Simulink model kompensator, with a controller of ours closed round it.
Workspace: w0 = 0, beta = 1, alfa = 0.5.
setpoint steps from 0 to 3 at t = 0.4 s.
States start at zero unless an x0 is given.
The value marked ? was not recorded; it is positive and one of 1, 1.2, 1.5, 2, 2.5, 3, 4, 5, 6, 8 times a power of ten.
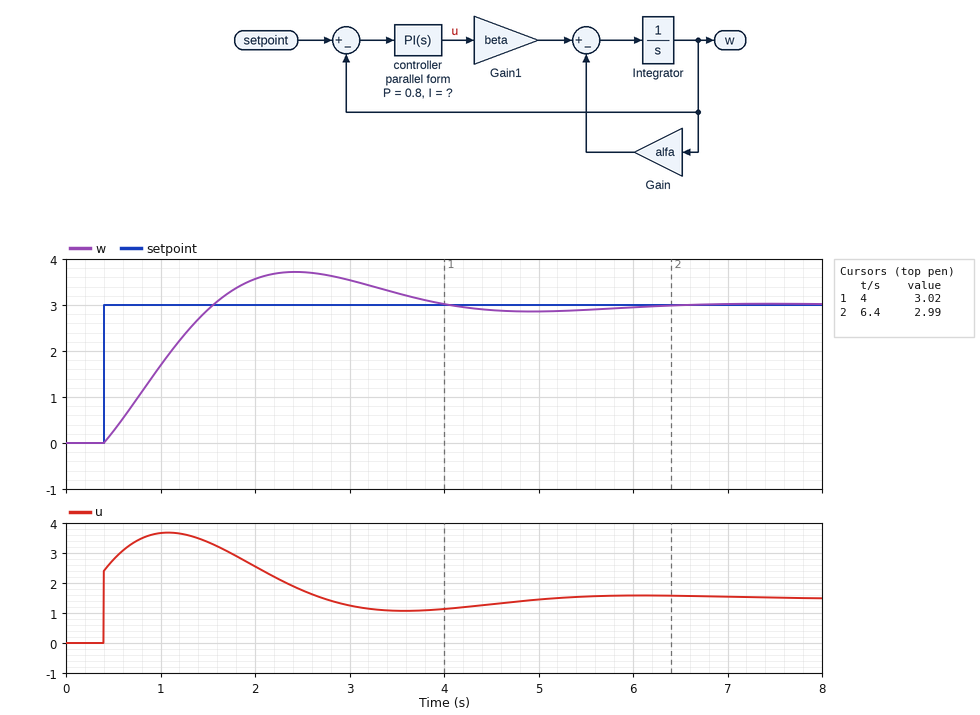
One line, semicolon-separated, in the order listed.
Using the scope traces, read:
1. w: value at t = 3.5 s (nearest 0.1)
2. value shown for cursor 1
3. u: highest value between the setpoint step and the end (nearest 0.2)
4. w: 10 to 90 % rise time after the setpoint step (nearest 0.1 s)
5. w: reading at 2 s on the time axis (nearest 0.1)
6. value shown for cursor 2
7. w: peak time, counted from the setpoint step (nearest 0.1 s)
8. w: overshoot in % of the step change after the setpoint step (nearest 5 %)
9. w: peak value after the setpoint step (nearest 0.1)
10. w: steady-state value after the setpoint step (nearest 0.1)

3.3; 3.02; 3.6; 0.9 s; 3.6; 2.99; 2.0 s; 25 %; 3.7; 3.0
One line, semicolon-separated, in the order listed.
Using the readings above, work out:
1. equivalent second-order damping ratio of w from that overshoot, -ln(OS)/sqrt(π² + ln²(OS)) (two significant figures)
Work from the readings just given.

0.40
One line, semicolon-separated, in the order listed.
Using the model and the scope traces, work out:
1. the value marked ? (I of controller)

2
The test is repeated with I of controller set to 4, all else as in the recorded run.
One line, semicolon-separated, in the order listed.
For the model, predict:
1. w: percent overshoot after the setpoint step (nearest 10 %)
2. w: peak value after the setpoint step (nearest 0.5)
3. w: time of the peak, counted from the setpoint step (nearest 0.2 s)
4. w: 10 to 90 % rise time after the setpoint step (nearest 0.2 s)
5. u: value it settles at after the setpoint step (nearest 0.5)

40 %; 4.0; 1.4 s; 0.6 s; 1.5
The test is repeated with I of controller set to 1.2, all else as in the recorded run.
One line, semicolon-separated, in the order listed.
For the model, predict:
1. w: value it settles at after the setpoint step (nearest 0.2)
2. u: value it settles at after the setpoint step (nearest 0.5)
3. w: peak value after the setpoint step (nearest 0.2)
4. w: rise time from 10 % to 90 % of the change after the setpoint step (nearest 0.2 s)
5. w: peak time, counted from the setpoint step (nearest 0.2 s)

3.0; 1.5; 3.4; 1.2 s; 2.6 s
